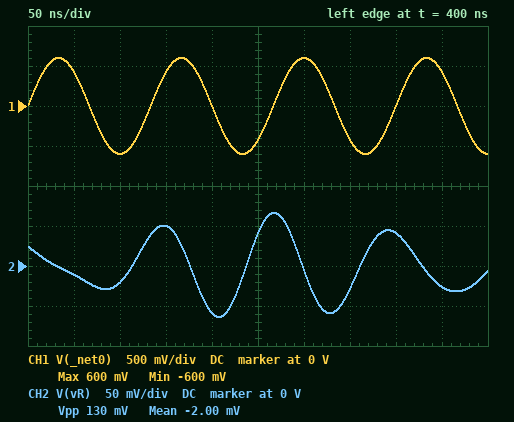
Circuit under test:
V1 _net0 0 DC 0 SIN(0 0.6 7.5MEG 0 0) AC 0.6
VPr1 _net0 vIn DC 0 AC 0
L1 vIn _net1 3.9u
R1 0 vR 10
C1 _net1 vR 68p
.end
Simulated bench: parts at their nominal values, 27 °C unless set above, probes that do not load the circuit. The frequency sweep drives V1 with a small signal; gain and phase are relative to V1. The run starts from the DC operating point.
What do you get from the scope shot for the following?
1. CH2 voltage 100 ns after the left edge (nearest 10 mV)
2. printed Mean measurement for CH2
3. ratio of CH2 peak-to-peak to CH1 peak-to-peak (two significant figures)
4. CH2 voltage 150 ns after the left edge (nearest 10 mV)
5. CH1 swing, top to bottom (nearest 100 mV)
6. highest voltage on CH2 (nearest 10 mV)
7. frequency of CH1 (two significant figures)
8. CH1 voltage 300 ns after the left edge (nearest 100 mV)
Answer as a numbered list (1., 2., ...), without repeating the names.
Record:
1. -20 mV
2. -2.00 mV
3. 0.11
4. 50 mV
5. 1.2 V
6. 70 mV
7. 7.5 MHz
8. 600 mV
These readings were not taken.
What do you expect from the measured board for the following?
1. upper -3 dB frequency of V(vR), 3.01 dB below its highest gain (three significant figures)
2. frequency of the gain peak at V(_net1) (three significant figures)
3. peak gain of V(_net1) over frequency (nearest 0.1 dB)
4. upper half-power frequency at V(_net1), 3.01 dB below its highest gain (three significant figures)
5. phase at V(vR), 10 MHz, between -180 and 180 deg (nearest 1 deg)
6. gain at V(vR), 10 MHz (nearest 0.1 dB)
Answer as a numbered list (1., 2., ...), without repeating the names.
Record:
1. 9.98 MHz
2. 9.77 MHz
3. 27.6 dB
4. 9.97 MHz
5. -48 deg
6. -3.4 dB
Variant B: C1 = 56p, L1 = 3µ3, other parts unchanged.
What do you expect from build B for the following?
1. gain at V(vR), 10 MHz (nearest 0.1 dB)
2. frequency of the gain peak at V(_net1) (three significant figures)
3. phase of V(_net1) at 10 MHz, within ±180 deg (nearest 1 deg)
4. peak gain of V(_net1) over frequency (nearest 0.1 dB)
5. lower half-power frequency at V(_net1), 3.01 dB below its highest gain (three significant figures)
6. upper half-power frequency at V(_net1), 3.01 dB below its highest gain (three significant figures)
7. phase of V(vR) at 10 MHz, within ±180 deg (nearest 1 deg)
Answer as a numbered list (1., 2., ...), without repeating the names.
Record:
1. -17.8 dB
2. 11.7 MHz
3. -5 deg
4. 27.7 dB
5. 11.5 MHz
6. 11.9 MHz
7. 83 deg
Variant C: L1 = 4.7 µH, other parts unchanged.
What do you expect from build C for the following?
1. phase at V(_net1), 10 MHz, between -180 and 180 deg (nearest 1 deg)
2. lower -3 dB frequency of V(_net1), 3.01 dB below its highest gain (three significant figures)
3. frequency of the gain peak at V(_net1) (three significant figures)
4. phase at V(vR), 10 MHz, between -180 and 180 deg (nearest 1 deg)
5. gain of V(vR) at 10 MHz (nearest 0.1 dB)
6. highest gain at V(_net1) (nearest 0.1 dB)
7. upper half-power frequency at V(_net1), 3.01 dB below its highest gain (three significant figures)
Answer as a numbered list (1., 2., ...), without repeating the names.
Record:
1. -168 deg
2. 8.73 MHz
3. 8.90 MHz
4. -81 deg
5. -15.9 dB
6. 28.4 dB
7. 9.07 MHz
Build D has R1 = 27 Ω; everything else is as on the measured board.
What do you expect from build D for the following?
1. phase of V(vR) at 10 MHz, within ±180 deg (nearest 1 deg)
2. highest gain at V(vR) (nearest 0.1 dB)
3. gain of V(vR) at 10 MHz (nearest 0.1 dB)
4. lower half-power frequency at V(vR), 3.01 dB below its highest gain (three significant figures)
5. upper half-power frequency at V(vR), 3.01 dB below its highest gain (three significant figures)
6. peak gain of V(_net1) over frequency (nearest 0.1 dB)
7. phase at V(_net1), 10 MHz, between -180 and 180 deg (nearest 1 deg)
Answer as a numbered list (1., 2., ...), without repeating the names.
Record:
1. -22 deg
2. 0 dB
3. -0.7 dB
4. 9.24 MHz
5. 10.3 MHz
6. 19.0 dB
7. -106 deg
